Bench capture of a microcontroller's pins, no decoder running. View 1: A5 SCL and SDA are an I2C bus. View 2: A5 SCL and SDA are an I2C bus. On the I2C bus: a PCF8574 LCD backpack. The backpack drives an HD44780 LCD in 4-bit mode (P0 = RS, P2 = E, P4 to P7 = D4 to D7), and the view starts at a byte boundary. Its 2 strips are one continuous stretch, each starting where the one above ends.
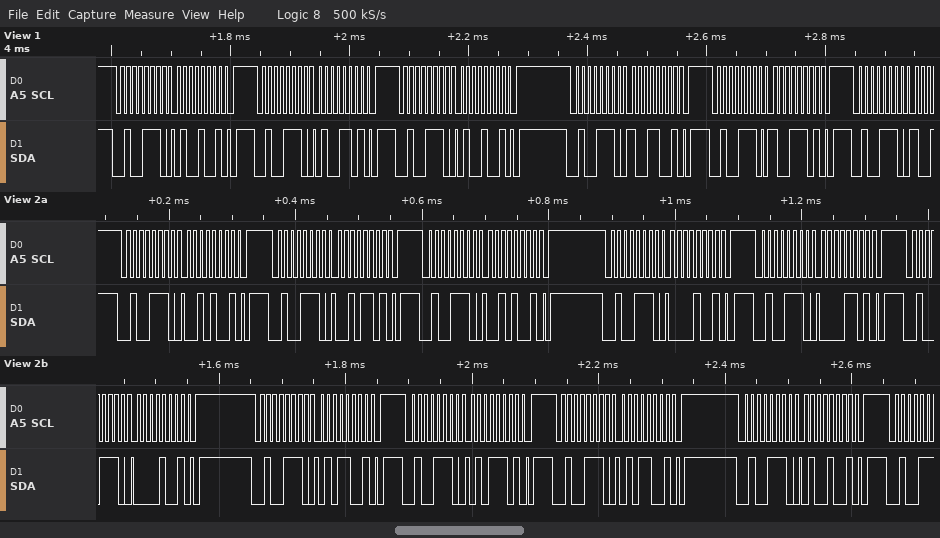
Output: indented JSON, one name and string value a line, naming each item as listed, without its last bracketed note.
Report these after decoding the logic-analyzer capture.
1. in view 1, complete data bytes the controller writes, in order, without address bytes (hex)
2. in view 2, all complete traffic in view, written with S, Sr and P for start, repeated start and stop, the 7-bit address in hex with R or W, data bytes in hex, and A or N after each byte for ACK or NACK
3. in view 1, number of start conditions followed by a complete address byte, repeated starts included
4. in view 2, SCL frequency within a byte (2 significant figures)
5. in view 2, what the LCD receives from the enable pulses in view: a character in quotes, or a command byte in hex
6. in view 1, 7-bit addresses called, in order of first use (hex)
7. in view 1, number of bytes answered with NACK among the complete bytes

{
  "in view 1, complete data bytes the controller writes, in order, without address bytes": "49 4D 49 99 9D",
  "in view 2, all complete traffic in view, written with S, Sr and P for start, repeated start and stop, the 7-bit address in hex with R or W, data bytes in hex, and A or N after each byte for ACK or NACK": "S 27W A 29 A P S 27W A 2D A P S 27W A 29 A P S 27W A 09 A P S 27W A 0D A P S 27W A 09 A P S 27W A 59 A P S 27W A 5D A P S 27W A 59 A P S 27W A 49 A P",
  "in view 1, number of start conditions followed by a complete address byte, repeated starts included": "6",
  "in view 2, SCL frequency within a byte": "100 kHz",
  "in view 2, what the LCD receives from the enable pulses in view: a character in quotes, or a command byte in hex": "' '",
  "in view 1, 7-bit addresses called, in order of first use": "0x27",
  "in view 1, number of bytes answered with NACK among the complete bytes": "0"
}
